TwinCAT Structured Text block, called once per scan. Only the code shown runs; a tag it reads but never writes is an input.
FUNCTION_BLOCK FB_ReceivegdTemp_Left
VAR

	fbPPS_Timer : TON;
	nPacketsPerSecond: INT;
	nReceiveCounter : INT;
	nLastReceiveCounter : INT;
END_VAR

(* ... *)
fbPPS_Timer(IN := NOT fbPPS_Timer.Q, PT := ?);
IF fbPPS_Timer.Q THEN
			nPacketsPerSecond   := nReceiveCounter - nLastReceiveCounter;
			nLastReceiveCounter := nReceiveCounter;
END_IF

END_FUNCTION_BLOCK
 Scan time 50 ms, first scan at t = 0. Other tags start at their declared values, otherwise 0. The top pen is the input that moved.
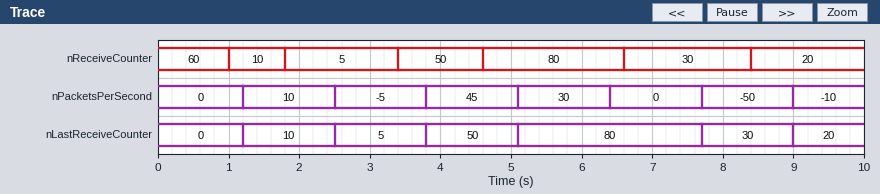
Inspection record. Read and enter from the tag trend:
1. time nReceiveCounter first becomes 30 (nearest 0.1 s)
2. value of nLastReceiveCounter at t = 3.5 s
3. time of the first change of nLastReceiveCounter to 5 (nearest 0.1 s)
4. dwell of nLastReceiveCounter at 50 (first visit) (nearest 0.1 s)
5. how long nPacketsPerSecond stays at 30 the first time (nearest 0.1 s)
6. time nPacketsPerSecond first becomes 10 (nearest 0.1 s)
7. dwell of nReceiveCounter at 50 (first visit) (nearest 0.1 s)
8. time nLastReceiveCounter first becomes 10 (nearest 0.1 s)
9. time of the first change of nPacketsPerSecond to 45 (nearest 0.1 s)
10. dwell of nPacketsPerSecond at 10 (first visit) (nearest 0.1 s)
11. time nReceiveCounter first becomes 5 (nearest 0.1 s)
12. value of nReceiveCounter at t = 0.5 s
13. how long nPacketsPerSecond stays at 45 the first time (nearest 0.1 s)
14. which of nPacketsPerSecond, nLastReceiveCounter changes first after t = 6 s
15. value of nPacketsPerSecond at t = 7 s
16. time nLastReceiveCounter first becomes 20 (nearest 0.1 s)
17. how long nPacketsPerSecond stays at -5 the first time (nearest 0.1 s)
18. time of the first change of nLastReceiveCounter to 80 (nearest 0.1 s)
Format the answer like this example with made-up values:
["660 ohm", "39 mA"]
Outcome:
["6.6 s", "5", "2.5 s", "1.3 s", "1.3 s", "1.2 s", "1.2 s", "1.2 s", "3.8 s", "1.3 s", "1.8 s", "60", "1.3 s", "nPacketsPerSecond", "0", "9.0 s", "1.3 s", "5.1 s"]
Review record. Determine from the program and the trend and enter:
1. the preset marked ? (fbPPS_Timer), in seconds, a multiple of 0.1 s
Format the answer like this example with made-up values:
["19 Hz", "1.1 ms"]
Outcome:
["1.2 s"]
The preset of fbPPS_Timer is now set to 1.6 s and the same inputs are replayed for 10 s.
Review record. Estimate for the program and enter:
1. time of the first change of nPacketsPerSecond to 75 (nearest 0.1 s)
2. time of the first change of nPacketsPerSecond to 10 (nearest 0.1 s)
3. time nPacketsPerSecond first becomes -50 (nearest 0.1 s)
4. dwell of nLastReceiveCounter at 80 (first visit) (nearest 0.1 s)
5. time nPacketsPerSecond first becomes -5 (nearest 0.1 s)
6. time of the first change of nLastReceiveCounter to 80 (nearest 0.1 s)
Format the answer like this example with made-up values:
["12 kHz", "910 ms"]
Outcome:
["5.0 s", "1.6 s", "6.7 s", "1.7 s", "3.3 s", "5.0 s"]
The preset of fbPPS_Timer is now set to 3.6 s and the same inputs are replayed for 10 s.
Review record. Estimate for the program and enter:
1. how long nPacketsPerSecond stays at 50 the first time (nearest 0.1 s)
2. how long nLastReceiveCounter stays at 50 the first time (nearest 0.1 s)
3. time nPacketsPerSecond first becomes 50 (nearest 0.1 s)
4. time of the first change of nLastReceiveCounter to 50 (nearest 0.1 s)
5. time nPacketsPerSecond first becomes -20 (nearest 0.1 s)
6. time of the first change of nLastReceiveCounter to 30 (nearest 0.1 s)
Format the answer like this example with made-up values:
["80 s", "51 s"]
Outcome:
["3.7 s", "3.7 s", "3.6 s", "3.6 s", "7.3 s", "7.3 s"]
